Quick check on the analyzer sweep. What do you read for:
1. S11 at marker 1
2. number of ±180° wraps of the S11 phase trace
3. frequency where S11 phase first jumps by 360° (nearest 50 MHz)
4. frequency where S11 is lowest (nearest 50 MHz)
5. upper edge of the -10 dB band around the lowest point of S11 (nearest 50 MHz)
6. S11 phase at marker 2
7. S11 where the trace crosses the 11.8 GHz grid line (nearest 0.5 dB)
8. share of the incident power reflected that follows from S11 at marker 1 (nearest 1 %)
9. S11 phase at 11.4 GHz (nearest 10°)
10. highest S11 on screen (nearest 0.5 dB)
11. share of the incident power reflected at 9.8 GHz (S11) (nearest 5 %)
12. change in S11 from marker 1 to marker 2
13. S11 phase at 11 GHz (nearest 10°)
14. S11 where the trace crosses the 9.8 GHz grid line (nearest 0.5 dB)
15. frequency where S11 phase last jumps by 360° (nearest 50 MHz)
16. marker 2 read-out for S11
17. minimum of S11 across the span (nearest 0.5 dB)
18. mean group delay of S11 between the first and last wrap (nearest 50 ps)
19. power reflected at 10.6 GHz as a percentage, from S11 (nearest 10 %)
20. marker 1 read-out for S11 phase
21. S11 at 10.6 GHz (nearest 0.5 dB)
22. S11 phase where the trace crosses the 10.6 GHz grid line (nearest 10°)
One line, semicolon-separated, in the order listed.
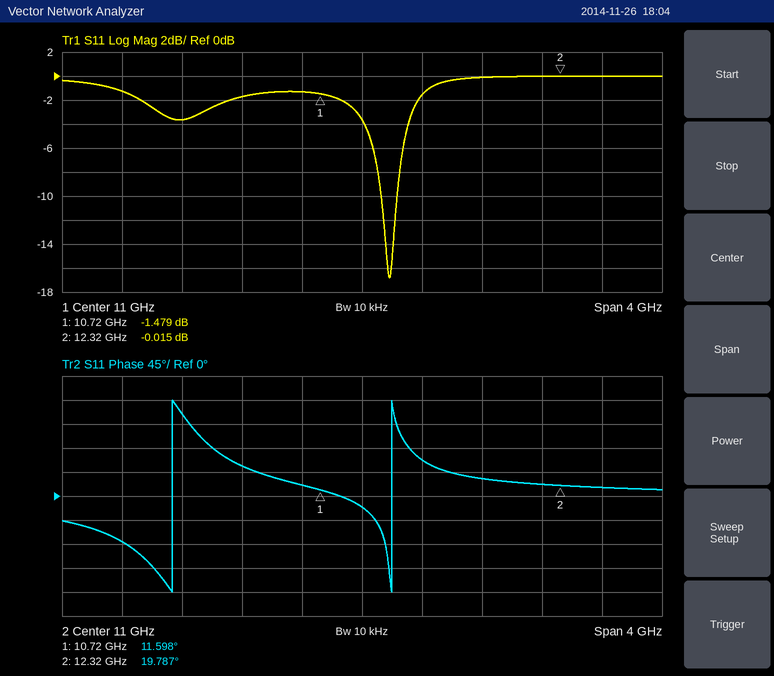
-1.479 dB; 2; 9.75 GHz; 11.20 GHz; 11.25 GHz; 19.787°; 0.0 dB; 71 %; 70°; 0.0 dB; 45 %; 1.464 dB; -20°; -3.5 dB; 11.20 GHz; -0.015 dB; -17.0 dB; 700 ps; 70 %; 11.598°; -1.5 dB; 20°
